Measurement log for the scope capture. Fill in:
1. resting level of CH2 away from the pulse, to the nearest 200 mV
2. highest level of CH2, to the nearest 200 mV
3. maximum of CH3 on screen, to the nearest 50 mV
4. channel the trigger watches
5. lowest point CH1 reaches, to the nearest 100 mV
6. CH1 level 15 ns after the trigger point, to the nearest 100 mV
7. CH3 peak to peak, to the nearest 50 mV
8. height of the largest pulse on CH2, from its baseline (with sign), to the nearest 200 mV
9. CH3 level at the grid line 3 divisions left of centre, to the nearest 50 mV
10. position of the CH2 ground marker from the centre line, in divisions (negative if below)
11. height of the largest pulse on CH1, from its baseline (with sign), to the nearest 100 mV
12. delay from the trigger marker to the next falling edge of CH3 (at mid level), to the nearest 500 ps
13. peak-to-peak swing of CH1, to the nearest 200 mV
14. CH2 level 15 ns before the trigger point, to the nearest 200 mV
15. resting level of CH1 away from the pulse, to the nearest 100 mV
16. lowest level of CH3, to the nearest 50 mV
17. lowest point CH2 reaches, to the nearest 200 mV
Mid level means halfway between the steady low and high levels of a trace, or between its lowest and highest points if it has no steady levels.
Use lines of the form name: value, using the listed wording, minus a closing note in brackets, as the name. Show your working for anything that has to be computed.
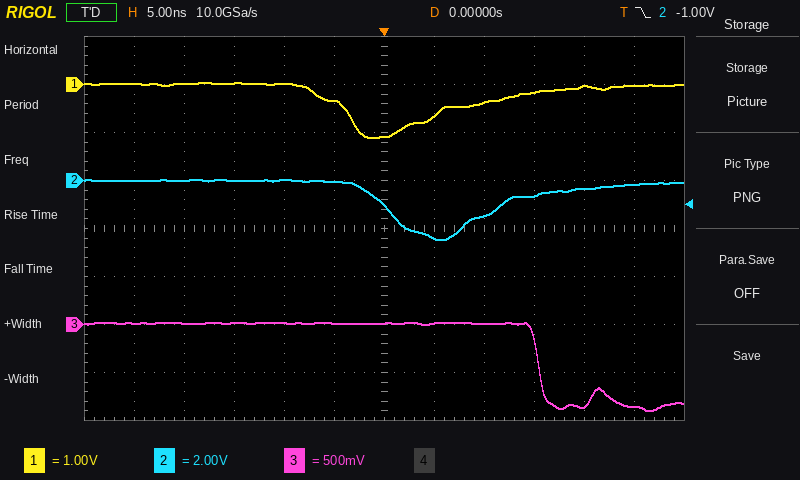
resting level of CH2 away from the pulse, to the nearest 200 mV: 0.0 V
highest level of CH2, to the nearest 200 mV: 0.0 V
maximum of CH3 on screen, to the nearest 50 mV: 0 mV
channel the trigger watches: CH2
lowest point CH1 reaches, to the nearest 100 mV: -1.1 V
CH1 level 15 ns after the trigger point, to the nearest 100 mV: -200 mV
CH3 peak to peak, to the nearest 50 mV: 0 mV − (-900 mV) = 900 mV
height of the largest pulse on CH2, from its baseline (with sign), to the nearest 200 mV: -2.4 V − (0.0 V) = -2.4 V
CH3 level at the grid line 3 divisions left of centre, to the nearest 50 mV: 0 mV
position of the CH2 ground marker from the centre line, in divisions: +1.0 div
height of the largest pulse on CH1, from its baseline (with sign), to the nearest 100 mV: -1.1 V − (0.0 V) = -1.1 V
delay from the trigger marker to the next falling edge of CH3 (at mid level), to the nearest 500 ps: 15.5 ns
peak-to-peak swing of CH1, to the nearest 200 mV: 1.2 V
CH2 level 15 ns before the trigger point, to the nearest 200 mV: 0.0 V
resting level of CH1 away from the pulse, to the nearest 100 mV: 0.0 V
lowest level of CH3, to the nearest 50 mV: -900 mV
lowest point CH2 reaches, to the nearest 200 mV: -2.4 V
